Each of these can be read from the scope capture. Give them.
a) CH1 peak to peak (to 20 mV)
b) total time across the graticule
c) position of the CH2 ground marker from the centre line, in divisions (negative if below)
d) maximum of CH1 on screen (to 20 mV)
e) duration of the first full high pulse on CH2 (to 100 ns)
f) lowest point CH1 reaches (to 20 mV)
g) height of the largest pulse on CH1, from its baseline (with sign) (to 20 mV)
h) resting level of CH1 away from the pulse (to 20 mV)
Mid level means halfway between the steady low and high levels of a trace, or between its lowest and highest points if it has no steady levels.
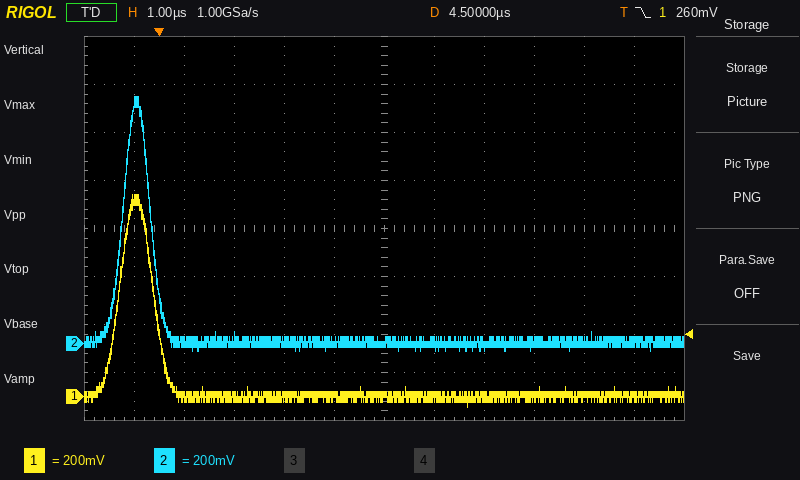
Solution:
880 mV
12 µs
-2.4 div
840 mV
600 ns
-40 mV
+840 mV
0 mV
